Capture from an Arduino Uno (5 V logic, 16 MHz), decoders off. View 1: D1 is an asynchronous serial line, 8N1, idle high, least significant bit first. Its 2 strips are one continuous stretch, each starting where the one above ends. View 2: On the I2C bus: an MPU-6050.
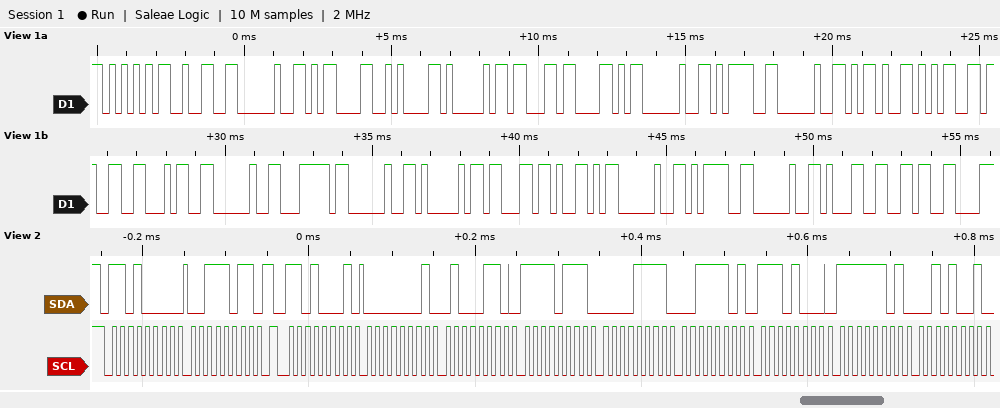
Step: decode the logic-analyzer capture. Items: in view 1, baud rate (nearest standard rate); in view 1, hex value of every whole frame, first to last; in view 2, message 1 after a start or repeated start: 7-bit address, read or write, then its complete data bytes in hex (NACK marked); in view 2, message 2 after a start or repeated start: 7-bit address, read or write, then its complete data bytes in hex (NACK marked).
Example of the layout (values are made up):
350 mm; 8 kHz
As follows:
4800 baud; 55 32 20 0D 0A 41 63 58 20 3D 20 2D 35 33 34 20 7C 20 41 63 59 20 3D 20 31 36; 0x68 write: 3B; 0x68 read: 01 46 F7 0F 3D E8 FD 29
